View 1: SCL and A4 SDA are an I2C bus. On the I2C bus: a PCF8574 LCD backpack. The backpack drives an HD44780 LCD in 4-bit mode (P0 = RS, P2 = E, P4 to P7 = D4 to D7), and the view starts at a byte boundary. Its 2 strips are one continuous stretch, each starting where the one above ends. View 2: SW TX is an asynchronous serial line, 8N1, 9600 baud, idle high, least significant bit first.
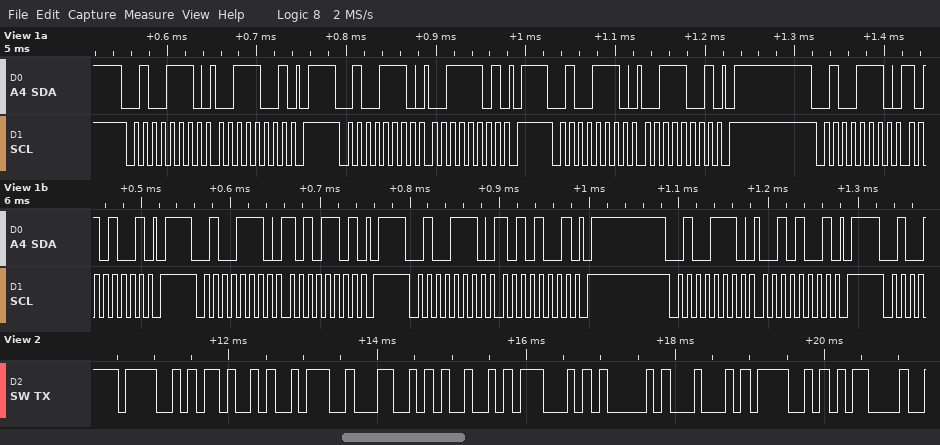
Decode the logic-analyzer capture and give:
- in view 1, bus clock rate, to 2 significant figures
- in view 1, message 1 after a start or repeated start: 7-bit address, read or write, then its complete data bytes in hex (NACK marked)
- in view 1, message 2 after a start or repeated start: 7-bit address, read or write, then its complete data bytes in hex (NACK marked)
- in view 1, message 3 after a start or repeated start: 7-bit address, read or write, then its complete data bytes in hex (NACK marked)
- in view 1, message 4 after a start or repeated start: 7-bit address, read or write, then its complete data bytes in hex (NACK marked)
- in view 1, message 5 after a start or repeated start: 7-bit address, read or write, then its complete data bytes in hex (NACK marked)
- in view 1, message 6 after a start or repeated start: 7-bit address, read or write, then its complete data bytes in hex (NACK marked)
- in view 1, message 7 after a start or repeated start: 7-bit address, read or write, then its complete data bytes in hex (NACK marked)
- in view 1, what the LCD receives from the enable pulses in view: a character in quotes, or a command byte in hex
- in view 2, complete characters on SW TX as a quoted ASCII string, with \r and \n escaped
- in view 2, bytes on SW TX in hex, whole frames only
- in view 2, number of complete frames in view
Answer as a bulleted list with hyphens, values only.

- 100 kHz
- 0x27 write: 39
- 0x27 write: 3D
- 0x27 write: 39
- 0x27 write: A9
- 0x27 write: AD
- 0x27 write: A9
- 0x27 write: 29
- ':'
- "OK:LIGADO\r"
- 4F 4B 3A 4C 49 47 41 44 4F 0D
- 10
